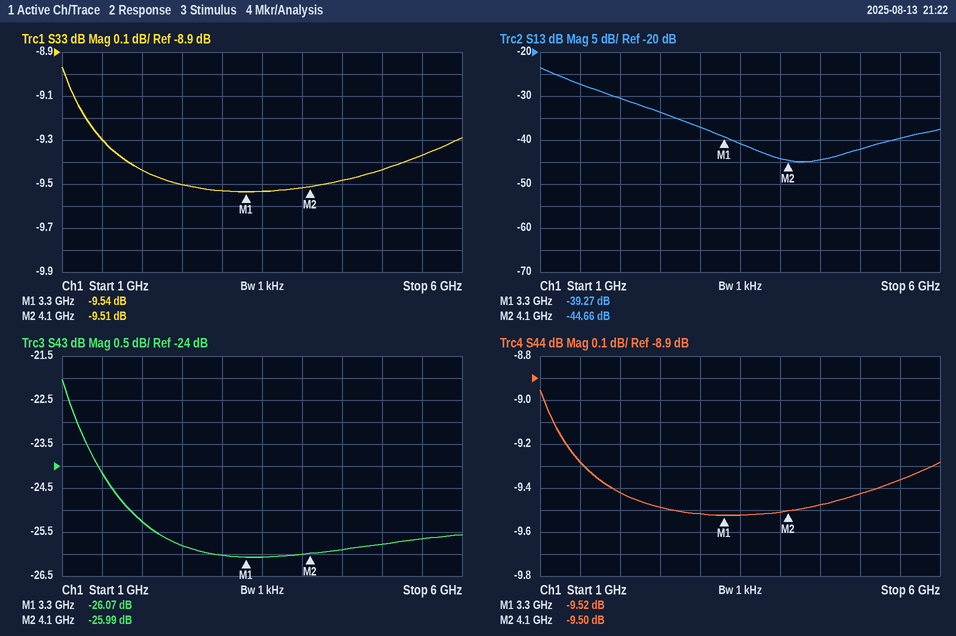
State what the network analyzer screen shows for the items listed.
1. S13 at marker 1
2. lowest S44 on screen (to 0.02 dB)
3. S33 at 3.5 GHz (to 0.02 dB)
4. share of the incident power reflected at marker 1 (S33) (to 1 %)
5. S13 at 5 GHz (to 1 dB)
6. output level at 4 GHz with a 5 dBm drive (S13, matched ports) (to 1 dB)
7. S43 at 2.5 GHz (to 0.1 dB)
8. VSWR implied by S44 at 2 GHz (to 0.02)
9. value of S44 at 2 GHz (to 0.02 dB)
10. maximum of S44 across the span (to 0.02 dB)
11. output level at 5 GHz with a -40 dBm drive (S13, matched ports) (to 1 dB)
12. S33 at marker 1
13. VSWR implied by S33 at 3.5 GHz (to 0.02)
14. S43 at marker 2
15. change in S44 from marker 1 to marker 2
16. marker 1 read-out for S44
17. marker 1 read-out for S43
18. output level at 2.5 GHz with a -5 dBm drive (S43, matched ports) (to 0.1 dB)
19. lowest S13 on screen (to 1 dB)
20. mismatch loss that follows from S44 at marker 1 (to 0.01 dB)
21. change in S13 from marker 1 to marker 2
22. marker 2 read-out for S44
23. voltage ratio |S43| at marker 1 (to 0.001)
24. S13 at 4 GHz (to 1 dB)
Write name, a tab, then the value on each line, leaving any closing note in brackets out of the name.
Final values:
S13 at marker 1	-39.27 dB
lowest S44 on screen	-9.52 dB
S33 at 3.5 GHz	-9.54 dB
share of the incident power reflected at marker 1 (S33)	11 %
S13 at 5 GHz	-42 dB
output level at 4 GHz with a 5 dBm drive (S13, matched ports)	-39 dBm
S43 at 2.5 GHz	-25.8 dB
VSWR implied by S44 at 2 GHz	2.02
value of S44 at 2 GHz	-9.42 dB
maximum of S44 across the span	-8.96 dB
output level at 5 GHz with a -40 dBm drive (S13, matched ports)	-82 dBm
S33 at marker 1	-9.54 dB
VSWR implied by S33 at 3.5 GHz	2.00
S43 at marker 2	-25.99 dB
change in S44 from marker 1 to marker 2	0.02 dB
marker 1 read-out for S44	-9.52 dB
marker 1 read-out for S43	-26.07 dB
output level at 2.5 GHz with a -5 dBm drive (S43, matched ports)	-30.8 dBm
lowest S13 on screen	-45 dB
mismatch loss that follows from S44 at marker 1	0.51 dB
change in S13 from marker 1 to marker 2	-5.39 dB
marker 2 read-out for S44	-9.50 dB
voltage ratio |S43| at marker 1	0.050
S13 at 4 GHz	-44 dB
